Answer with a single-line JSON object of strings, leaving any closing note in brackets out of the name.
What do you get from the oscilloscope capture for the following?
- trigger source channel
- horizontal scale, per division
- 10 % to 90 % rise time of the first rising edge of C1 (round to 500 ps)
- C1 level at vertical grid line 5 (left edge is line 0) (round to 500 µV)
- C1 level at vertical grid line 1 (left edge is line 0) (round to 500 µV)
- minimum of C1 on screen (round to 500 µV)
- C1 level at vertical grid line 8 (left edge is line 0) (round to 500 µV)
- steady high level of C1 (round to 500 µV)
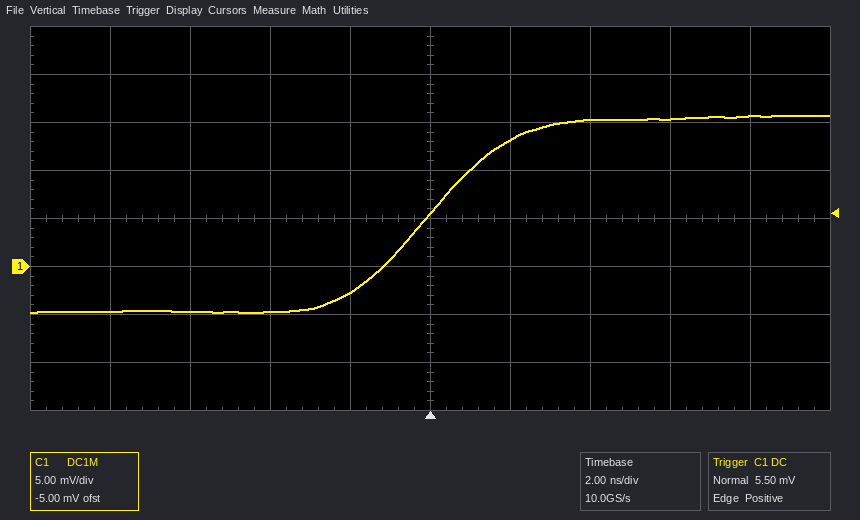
{"trigger source channel": "C1", "horizontal scale, per division": "2 ns", "10 % to 90 % rise time of the first rising edge of C1": "4.0 ns", "C1 level at vertical grid line 5 (left edge is line 0)": "5.5 mV", "C1 level at vertical grid line 1 (left edge is line 0)": "-4.5 mV", "minimum of C1 on screen": "-5.0 mV", "C1 level at vertical grid line 8 (left edge is line 0)": "15.5 mV", "steady high level of C1": "15.5 mV"}
